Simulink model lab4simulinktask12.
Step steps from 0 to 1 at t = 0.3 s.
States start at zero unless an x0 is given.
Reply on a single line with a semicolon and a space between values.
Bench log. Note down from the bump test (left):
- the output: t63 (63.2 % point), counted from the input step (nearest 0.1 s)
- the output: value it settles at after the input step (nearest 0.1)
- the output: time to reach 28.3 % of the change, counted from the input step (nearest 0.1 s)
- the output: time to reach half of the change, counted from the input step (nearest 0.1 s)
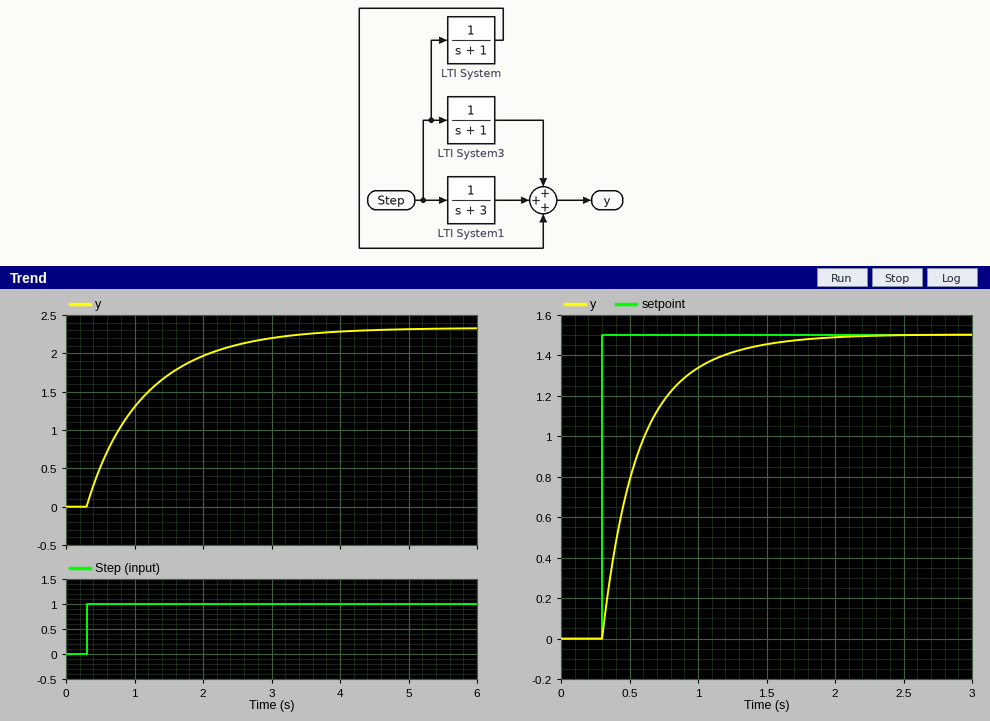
0.9 s; 2.3; 0.3 s; 0.6 s
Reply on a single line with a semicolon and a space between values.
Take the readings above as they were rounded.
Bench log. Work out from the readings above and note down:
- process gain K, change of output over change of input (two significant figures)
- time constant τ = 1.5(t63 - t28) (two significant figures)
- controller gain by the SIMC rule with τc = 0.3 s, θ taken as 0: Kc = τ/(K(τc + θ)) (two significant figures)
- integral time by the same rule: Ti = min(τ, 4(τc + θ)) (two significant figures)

2.3; 0.90 s; 1.3; 0.90 s
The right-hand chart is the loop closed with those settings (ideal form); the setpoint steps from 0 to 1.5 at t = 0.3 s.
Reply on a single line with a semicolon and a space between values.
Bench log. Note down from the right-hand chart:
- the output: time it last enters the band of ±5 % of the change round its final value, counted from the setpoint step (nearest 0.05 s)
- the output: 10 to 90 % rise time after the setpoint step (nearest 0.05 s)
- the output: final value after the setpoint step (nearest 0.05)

1.00 s; 0.70 s; 1.50
